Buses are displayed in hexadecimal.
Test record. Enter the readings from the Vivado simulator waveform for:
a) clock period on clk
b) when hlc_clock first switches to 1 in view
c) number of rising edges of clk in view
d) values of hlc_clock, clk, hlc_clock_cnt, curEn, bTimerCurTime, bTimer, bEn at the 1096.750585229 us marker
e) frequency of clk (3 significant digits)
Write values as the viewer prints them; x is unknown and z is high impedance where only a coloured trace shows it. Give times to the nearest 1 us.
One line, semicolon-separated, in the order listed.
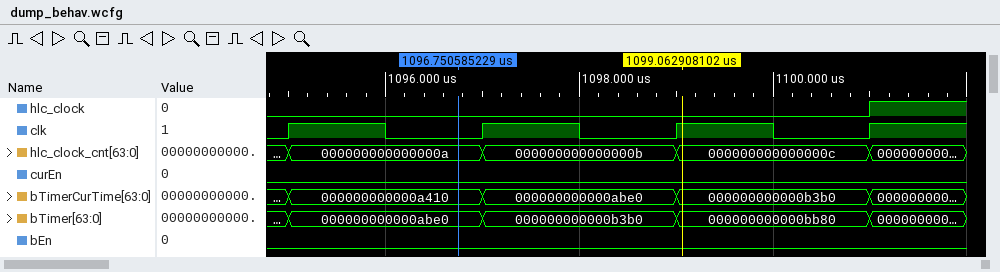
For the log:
2 us; 1101 us; 4; hlc_clock=0, clk=0, hlc_clock_cnt=000000000000000a, curEn=0, bTimerCurTime=000000000000a410, bTimer=000000000000abe0, bEn=0; 500 kHz
